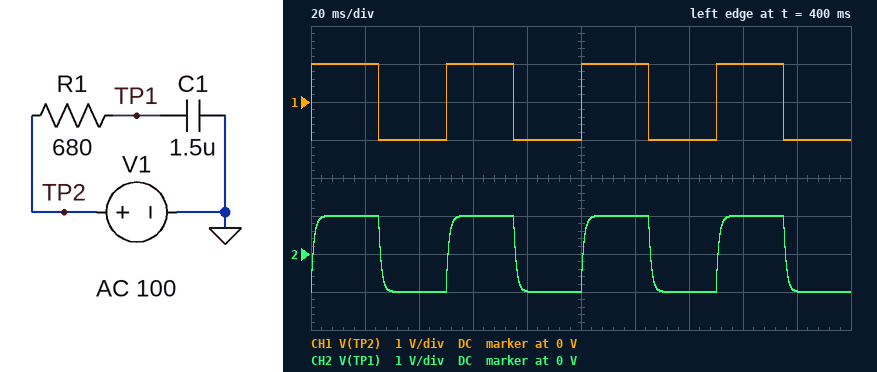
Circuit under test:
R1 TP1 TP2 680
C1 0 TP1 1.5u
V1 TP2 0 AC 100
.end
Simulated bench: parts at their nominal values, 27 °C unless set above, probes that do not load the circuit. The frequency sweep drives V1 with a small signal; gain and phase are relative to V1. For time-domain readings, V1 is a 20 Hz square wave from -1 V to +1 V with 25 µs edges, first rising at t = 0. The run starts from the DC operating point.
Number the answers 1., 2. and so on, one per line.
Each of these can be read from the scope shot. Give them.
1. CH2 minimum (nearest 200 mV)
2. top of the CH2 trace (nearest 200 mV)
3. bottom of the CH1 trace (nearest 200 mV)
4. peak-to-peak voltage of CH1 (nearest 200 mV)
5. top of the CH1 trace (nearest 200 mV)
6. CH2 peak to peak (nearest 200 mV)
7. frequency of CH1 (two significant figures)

1. -1.0 V
2. 1.0 V
3. -1.0 V
4. 2.0 V
5. 1.0 V
6. 2.0 V
7. 20 Hz
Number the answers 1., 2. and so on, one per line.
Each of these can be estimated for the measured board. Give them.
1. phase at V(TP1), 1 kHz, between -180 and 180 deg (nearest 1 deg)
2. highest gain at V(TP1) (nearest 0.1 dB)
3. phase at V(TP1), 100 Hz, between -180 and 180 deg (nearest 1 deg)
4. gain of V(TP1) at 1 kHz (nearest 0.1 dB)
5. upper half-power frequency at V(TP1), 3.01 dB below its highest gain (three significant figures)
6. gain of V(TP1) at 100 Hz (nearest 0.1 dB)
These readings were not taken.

1. -81 deg
2. 0 dB
3. -33 deg
4. -16.2 dB
5. 156 Hz
6. -1.5 dB
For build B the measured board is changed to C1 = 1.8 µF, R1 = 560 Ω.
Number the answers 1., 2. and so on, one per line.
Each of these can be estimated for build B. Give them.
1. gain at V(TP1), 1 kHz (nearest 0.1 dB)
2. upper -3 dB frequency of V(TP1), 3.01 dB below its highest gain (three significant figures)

1. -16.1 dB
2. 158 Hz
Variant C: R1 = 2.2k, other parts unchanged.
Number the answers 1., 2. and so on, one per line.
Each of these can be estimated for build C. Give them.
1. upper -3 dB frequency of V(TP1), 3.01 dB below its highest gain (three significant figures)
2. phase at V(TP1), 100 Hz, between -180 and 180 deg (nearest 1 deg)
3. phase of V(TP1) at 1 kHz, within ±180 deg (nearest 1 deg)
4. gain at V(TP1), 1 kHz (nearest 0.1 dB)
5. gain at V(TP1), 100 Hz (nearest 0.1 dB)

1. 48.2 Hz
2. -64 deg
3. -87 deg
4. -26.3 dB
5. -7.2 dB
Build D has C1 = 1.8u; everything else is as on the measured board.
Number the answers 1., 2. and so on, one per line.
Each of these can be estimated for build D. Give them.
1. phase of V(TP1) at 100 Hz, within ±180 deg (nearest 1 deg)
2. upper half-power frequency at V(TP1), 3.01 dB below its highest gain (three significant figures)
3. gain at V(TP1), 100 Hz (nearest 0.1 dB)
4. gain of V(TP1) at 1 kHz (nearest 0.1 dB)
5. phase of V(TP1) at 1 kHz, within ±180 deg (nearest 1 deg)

1. -38 deg
2. 130 Hz
3. -2.0 dB
4. -17.8 dB
5. -83 deg
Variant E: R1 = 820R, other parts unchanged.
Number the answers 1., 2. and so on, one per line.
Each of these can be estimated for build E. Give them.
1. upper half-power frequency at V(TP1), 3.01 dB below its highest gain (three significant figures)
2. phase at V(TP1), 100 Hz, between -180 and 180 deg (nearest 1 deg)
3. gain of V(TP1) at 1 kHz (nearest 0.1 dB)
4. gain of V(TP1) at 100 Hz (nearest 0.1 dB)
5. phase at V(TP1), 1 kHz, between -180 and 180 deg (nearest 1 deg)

1. 129 Hz
2. -38 deg
3. -17.8 dB
4. -2.0 dB
5. -83 deg
